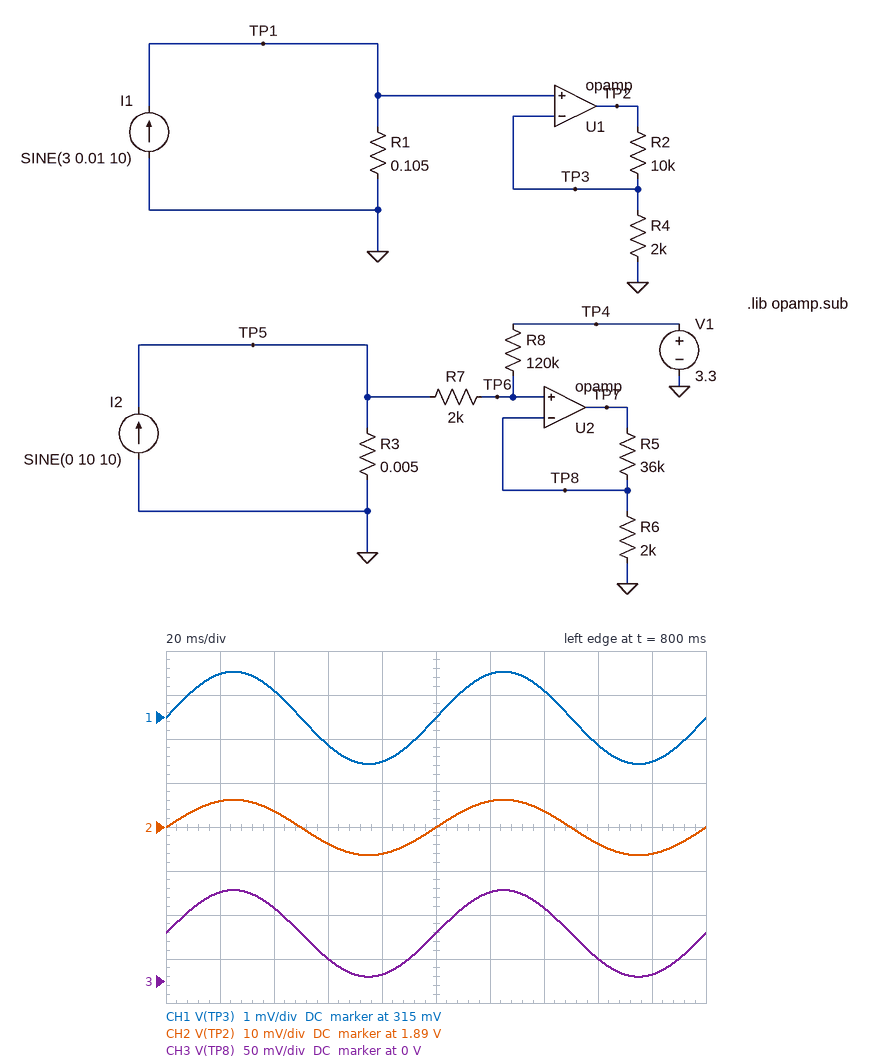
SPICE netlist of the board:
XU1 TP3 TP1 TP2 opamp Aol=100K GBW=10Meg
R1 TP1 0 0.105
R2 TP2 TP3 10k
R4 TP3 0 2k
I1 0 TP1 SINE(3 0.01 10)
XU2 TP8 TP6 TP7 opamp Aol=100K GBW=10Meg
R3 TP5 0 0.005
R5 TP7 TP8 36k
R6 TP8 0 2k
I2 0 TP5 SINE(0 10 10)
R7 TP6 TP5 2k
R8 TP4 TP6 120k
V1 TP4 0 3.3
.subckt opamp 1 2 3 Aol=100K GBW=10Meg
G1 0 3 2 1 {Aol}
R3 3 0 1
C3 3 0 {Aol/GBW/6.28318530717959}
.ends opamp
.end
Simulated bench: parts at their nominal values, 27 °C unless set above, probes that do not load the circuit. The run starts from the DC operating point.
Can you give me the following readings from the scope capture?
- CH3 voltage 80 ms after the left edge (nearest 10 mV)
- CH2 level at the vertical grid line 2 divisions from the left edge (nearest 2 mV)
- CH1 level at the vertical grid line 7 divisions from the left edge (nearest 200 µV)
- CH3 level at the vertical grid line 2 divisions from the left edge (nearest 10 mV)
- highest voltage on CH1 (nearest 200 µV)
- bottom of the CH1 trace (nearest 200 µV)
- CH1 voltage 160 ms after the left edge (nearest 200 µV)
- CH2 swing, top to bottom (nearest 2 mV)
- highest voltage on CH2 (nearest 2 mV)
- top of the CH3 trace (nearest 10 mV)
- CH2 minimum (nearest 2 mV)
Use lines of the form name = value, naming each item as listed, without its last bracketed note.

CH3 voltage 80 ms after the left edge = 10 mV
CH2 level at the vertical grid line 2 divisions from the left edge = 1.894 V
CH1 level at the vertical grid line 7 divisions from the left edge = 315.6 mV
CH3 level at the vertical grid line 2 divisions from the left edge = 80 mV
highest voltage on CH1 = 316.0 mV
bottom of the CH1 trace = 314.0 mV
CH1 voltage 160 ms after the left edge = 314.4 mV
CH2 swing, top to bottom = 12 mV
highest voltage on CH2 = 1.896 V
top of the CH3 trace = 100 mV
CH2 minimum = 1.884 V
